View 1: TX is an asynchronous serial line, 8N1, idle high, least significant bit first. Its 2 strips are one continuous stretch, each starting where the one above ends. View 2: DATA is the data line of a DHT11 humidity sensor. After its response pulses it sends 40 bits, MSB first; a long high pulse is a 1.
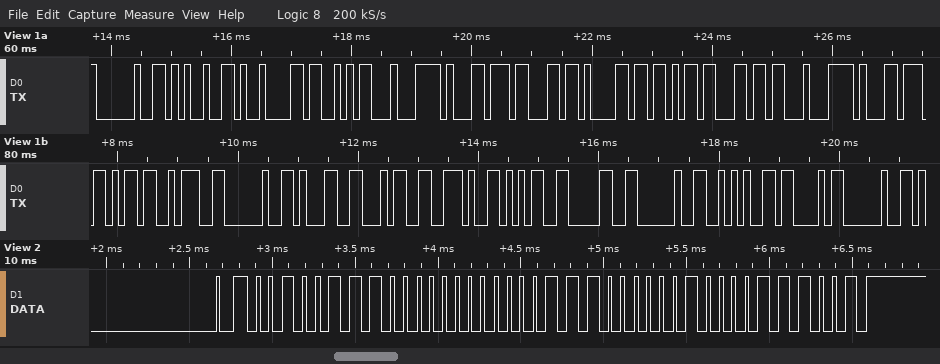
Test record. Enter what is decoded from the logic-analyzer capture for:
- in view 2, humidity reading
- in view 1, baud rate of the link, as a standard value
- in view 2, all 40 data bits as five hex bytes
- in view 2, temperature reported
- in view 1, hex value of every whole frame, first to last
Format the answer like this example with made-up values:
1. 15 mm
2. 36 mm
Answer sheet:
1. 39 %
2. 9600 baud
3. 27 00 0E 04 39
4. 14.4 °C
5. 20 25 09 53 C4 B1 63 61 6B 6C C4 B1 6B 3A 20 31 34 2E 35 30 20 2A 43 20
